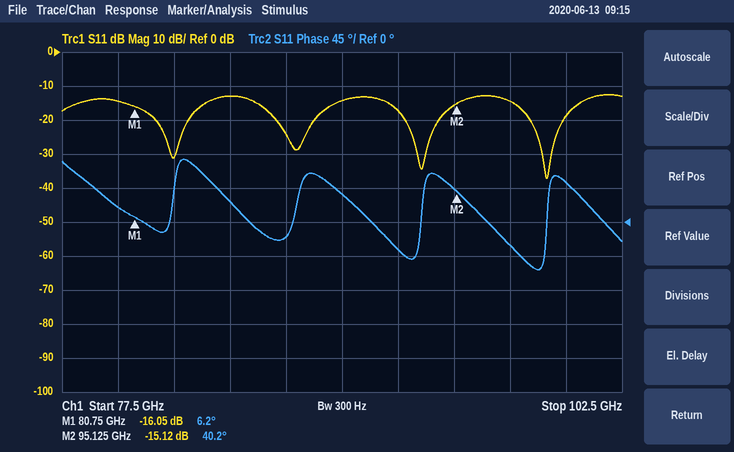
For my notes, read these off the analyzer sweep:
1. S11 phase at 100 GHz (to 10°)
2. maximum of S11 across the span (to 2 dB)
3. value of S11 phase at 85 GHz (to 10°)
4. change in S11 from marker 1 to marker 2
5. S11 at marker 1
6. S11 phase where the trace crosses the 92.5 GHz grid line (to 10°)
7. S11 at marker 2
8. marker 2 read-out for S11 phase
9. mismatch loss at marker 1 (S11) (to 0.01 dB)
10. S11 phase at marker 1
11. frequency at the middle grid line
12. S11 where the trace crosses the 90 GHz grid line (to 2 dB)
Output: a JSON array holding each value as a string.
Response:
["50°", "-12 dB", "30°", "0.93 dB", "-16.05 dB", "-40°", "-15.12 dB", "40.2°", "0.11 dB", "6.2°", "90 GHz", "-14 dB"]
